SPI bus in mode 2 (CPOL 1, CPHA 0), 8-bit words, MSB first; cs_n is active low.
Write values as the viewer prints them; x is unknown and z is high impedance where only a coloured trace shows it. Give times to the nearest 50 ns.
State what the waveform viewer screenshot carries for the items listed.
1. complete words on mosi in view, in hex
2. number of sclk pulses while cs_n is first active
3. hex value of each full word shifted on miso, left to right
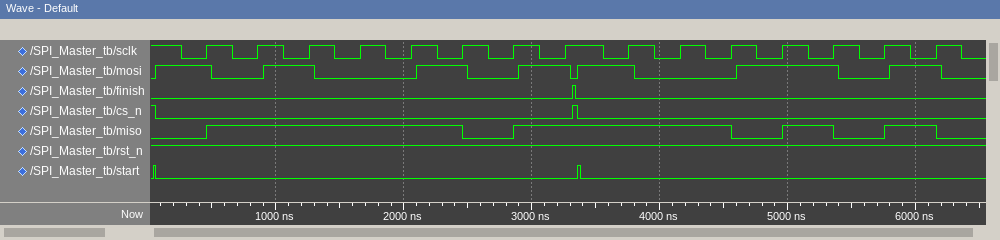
A5, 9A
8
7D, EA
